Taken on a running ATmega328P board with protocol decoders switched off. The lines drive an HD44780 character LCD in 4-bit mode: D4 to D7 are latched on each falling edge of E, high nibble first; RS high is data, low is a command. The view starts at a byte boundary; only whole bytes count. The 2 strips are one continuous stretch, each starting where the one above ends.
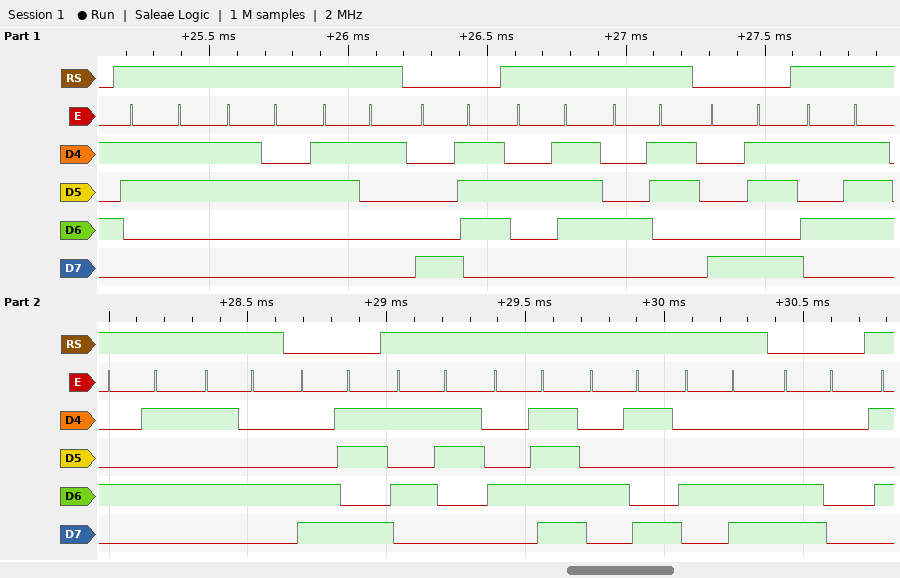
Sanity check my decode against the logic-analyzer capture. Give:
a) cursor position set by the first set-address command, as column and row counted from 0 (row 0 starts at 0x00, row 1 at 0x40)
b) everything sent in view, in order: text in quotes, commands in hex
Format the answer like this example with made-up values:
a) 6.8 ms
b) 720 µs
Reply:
a) column 7, row 0
b) "321" 0x87 "'C" 0x8B "WET" 0xCB "SOIL" 0xC0
